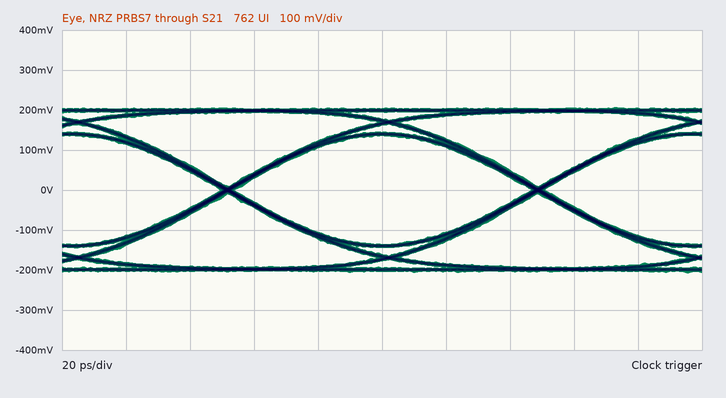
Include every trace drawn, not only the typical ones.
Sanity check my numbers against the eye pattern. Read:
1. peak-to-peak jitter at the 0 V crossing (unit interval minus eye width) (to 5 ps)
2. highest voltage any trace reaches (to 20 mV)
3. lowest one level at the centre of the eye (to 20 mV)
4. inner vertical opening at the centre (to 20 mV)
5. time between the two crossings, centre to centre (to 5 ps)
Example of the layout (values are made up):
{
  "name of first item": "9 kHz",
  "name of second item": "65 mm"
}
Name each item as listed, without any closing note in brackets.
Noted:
{
  "peak-to-peak jitter at the 0 V crossing (unit interval minus eye width)": "5 ps",
  "highest voltage any trace reaches": "200 mV",
  "lowest one level at the centre of the eye": "140 mV",
  "inner vertical opening at the centre": "280 mV",
  "time between the two crossings, centre to centre": "95 ps"
}
